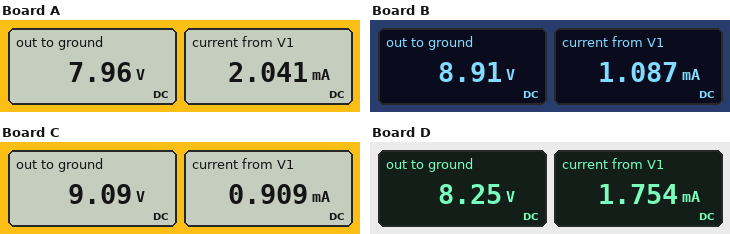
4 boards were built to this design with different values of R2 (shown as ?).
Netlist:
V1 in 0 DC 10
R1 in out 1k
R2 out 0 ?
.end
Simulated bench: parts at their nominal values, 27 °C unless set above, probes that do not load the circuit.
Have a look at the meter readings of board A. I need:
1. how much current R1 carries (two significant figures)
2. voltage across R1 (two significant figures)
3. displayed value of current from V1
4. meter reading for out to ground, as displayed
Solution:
2.0 mA
2.0 V
2.041 mA
7.96 V
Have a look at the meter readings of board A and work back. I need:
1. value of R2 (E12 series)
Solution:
3.9 kΩ
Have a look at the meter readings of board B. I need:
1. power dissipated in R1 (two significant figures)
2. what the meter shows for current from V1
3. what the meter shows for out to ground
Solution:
1.2 mW
1.087 mA
8.91 V
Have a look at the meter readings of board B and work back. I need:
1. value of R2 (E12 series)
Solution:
8.2 kΩ
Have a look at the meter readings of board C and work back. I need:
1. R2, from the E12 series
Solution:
10 kΩ
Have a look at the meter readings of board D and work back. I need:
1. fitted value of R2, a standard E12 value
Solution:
4.7 kΩ
